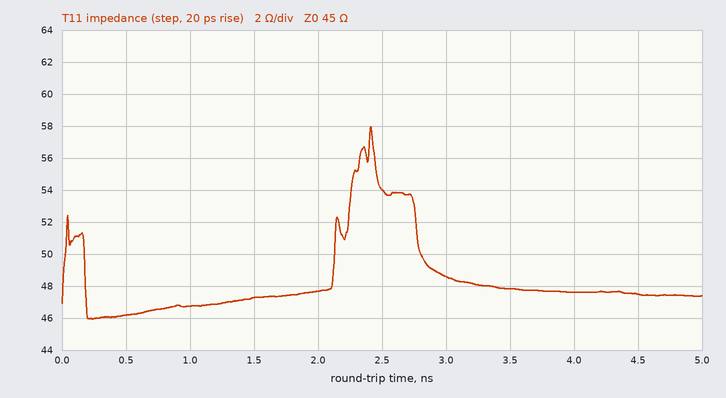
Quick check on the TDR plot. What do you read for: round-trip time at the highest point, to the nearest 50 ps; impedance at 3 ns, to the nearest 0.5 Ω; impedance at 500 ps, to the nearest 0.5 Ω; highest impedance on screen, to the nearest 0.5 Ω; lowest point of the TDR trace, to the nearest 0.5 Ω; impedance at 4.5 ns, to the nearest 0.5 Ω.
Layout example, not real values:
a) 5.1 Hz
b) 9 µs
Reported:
a) 2.40 ns
b) 48.5 Ω
c) 46.0 Ω
d) 58.0 Ω
e) 46.0 Ω
f) 47.5 Ω
